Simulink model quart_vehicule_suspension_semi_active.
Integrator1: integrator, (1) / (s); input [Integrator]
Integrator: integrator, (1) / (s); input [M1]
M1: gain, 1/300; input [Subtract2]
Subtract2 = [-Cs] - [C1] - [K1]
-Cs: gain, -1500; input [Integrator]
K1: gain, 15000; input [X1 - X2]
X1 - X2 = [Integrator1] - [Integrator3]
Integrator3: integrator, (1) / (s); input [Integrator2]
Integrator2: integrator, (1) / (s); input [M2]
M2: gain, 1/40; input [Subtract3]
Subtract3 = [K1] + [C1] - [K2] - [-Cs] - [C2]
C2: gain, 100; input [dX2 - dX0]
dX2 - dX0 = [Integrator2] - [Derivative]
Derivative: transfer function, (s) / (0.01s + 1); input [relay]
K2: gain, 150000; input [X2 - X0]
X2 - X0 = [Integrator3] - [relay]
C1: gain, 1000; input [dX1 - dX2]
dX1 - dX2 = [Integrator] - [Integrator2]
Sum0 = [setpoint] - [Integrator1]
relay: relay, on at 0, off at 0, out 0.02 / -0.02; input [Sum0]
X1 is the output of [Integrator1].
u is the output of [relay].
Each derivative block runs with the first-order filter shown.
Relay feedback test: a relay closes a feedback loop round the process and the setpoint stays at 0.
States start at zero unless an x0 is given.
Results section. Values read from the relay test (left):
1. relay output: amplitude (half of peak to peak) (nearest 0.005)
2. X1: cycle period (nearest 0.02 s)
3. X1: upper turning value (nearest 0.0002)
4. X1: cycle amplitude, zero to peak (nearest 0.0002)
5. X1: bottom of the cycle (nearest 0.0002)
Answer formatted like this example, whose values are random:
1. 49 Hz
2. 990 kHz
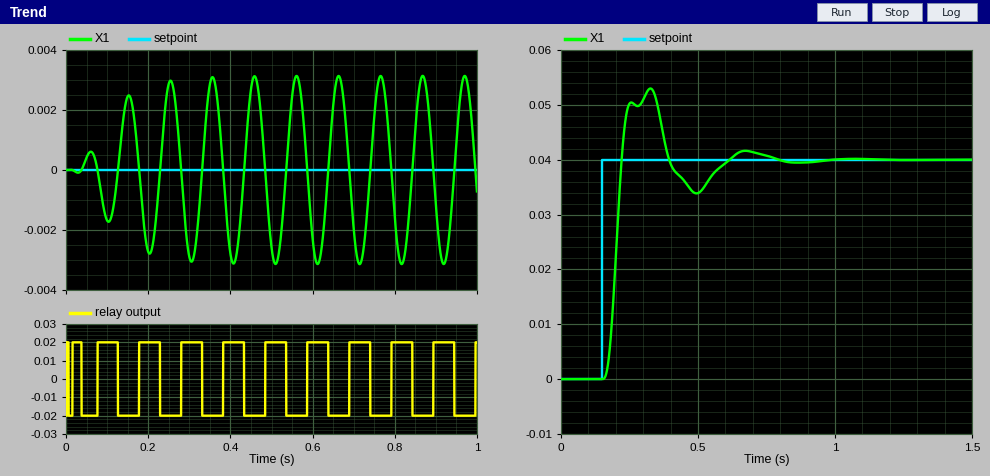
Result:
1. 0.020
2. 0.10 s
3. 0.0032
4. 0.0032
5. -0.0032
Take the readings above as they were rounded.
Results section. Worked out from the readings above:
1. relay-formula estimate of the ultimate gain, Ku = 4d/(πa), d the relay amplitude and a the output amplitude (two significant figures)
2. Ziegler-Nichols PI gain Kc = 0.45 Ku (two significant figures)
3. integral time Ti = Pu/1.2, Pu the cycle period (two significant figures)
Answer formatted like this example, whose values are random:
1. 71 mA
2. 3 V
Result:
1. 8.0
2. 3.6
3. 0.083 s
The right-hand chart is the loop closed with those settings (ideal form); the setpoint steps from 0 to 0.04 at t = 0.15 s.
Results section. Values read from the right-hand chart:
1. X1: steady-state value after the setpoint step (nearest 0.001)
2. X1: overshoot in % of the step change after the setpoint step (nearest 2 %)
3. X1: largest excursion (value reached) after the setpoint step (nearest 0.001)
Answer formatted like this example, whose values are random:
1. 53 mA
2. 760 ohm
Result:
1. 0.040
2. 32 %
3. 0.053
